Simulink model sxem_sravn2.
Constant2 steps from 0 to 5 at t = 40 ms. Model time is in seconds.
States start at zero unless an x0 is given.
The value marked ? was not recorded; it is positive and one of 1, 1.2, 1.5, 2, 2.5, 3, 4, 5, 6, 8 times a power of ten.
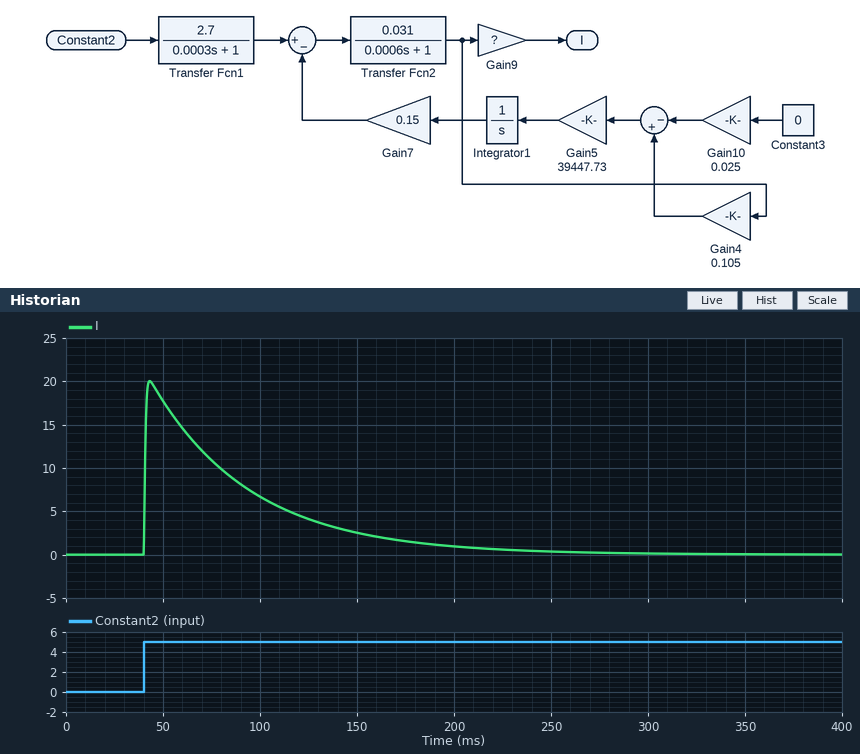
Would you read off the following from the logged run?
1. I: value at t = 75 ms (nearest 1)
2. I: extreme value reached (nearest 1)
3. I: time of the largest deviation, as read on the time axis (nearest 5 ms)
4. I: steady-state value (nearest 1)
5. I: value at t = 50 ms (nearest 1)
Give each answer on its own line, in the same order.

11
20
45 ms
0
18
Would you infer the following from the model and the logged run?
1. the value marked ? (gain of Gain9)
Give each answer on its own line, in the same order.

50
